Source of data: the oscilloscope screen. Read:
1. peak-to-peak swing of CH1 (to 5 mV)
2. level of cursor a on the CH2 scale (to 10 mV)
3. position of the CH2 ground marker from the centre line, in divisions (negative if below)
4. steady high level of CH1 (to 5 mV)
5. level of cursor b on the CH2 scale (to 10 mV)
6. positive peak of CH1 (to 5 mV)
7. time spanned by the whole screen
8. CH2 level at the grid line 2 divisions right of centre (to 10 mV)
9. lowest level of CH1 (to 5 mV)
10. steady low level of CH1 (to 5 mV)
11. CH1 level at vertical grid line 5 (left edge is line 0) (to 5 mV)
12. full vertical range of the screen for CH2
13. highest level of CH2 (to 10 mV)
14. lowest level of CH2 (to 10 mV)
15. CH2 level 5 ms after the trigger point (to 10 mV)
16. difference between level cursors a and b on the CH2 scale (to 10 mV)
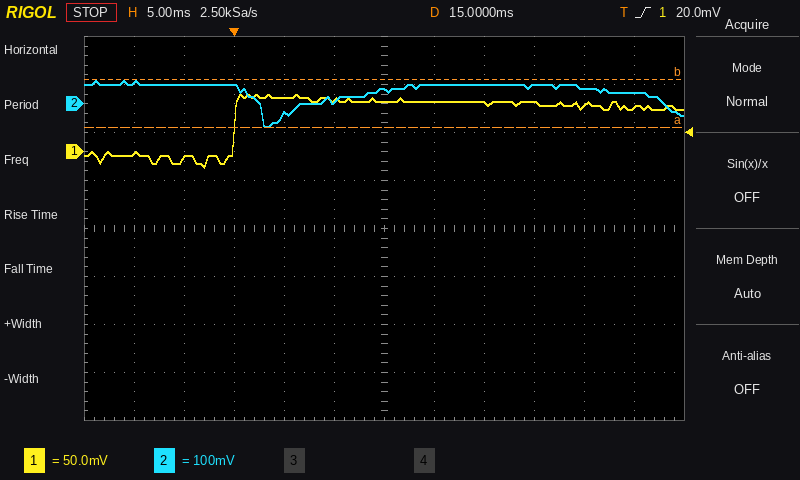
75 mV
-50 mV
+2.6 div
50 mV
50 mV
60 mV
60 ms
40 mV
-15 mV
-5 mV
55 mV
800 mV
50 mV
-50 mV
-20 mV
100 mV
